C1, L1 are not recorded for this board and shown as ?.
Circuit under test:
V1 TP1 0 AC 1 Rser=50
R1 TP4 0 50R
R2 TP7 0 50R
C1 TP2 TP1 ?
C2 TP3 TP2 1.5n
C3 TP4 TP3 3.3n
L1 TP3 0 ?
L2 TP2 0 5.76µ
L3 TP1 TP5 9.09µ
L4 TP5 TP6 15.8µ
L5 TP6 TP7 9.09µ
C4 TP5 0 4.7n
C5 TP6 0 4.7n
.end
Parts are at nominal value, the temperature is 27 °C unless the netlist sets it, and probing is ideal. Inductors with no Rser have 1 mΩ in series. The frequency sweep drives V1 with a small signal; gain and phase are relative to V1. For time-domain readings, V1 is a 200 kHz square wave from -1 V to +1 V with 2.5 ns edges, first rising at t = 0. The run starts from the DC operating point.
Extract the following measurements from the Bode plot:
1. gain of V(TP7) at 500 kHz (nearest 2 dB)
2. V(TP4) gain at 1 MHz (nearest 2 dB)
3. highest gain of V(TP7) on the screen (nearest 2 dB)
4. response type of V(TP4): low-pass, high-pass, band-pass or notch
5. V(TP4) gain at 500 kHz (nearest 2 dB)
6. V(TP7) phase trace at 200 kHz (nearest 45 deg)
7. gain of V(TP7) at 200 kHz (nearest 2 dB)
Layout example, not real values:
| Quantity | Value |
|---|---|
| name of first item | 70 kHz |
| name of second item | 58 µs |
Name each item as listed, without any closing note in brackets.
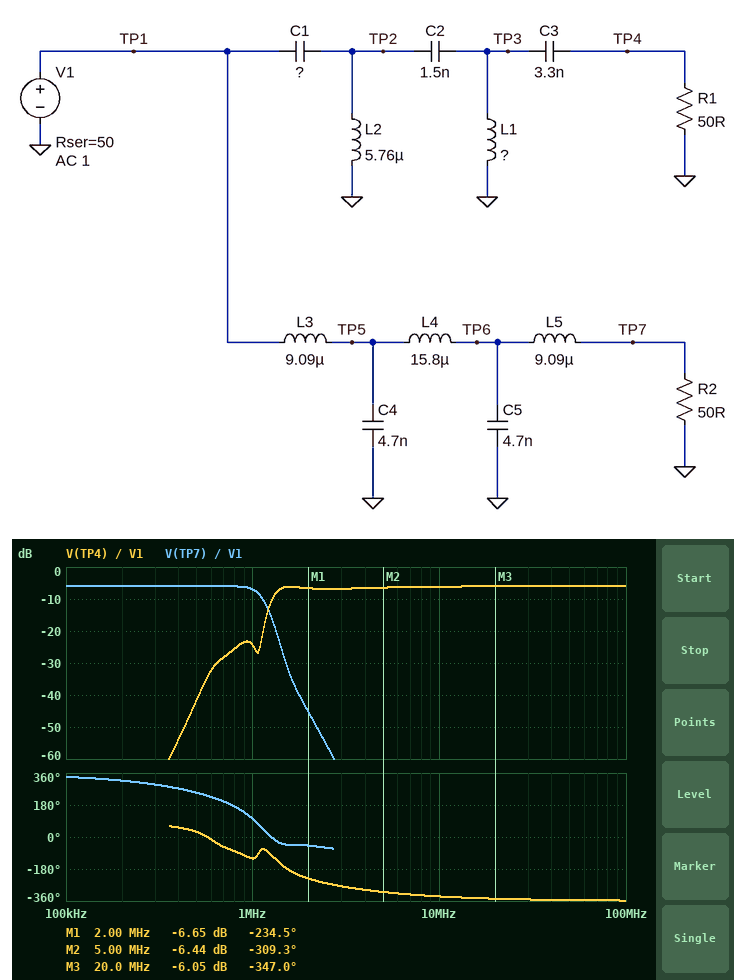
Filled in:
| Quantity | Value |
|---|---|
| gain of V(TP7) at 500 kHz | -6 dB |
| V(TP4) gain at 1 MHz | -24 dB |
| highest gain of V(TP7) on the screen | -6 dB |
| response type of V(TP4): low-pass, high-pass, band-pass or notch | high-pass |
| V(TP4) gain at 500 kHz | -42 dB |
| V(TP7) phase trace at 200 kHz | 315 deg |
| gain of V(TP7) at 200 kHz | -6 dB |
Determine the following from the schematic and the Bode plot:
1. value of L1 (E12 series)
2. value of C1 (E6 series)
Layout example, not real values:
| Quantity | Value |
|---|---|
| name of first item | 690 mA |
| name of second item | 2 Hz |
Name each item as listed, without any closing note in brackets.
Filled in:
| Quantity | Value |
|---|---|
| value of L1 | 15 µH |
| value of C1 | 1 nF |
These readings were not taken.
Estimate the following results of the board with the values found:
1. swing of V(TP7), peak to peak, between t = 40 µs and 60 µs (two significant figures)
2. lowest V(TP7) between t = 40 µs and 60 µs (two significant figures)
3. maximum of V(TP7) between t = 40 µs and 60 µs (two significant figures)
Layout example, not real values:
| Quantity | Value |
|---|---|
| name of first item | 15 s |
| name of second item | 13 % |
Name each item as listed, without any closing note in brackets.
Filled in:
| Quantity | Value |
|---|---|
| swing of V(TP7), peak to peak, between t = 40 µs and 60 µs | 1.3 V |
| lowest V(TP7) between t = 40 µs and 60 µs | -660 mV |
| maximum of V(TP7) between t = 40 µs and 60 µs | 660 mV |
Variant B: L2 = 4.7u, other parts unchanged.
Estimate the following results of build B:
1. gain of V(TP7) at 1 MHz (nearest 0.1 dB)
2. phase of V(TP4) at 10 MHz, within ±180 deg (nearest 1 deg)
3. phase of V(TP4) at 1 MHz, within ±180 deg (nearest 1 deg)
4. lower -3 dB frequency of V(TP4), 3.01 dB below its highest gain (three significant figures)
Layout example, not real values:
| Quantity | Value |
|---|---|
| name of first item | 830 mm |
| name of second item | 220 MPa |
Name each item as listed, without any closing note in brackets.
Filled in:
| Quantity | Value |
|---|---|
| gain of V(TP7) at 1 MHz | -6.9 dB |
| phase of V(TP4) at 10 MHz, within ±180 deg | 27 deg |
| phase of V(TP4) at 1 MHz, within ±180 deg | -116 deg |
| lower -3 dB frequency of V(TP4), 3.01 dB below its highest gain | 1.39 MHz |
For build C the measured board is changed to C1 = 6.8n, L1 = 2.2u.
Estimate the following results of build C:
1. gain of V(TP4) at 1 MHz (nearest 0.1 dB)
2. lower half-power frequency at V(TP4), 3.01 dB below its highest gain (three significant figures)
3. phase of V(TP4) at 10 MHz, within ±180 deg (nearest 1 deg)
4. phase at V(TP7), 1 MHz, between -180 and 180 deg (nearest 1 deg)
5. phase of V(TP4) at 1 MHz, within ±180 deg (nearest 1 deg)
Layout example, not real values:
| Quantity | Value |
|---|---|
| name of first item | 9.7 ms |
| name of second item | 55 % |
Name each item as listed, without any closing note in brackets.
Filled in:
| Quantity | Value |
|---|---|
| gain of V(TP4) at 1 MHz | -23.4 dB |
| lower half-power frequency at V(TP4), 3.01 dB below its highest gain | 1.60 MHz |
| phase of V(TP4) at 10 MHz, within ±180 deg | 27 deg |
| phase at V(TP7), 1 MHz, between -180 and 180 deg | 136 deg |
| phase of V(TP4) at 1 MHz, within ±180 deg | -130 deg |
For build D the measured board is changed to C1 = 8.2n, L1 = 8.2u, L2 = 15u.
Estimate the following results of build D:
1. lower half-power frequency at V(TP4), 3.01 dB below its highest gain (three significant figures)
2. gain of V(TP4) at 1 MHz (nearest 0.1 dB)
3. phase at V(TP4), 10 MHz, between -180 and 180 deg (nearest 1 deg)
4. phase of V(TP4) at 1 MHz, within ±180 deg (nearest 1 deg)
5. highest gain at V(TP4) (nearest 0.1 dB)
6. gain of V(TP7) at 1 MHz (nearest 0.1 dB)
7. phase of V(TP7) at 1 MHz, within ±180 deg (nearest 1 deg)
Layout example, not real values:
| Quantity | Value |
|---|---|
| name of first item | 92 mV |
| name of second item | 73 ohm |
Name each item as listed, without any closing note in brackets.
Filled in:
| Quantity | Value |
|---|---|
| lower half-power frequency at V(TP4), 3.01 dB below its highest gain | 1.32 MHz |
| gain of V(TP4) at 1 MHz | -14.1 dB |
| phase at V(TP4), 10 MHz, between -180 and 180 deg | 17 deg |
| phase of V(TP4) at 1 MHz, within ±180 deg | 135 deg |
| highest gain at V(TP4) | -6.0 dB |
| gain of V(TP7) at 1 MHz | -7.8 dB |
| phase of V(TP7) at 1 MHz, within ±180 deg | 111 deg |
